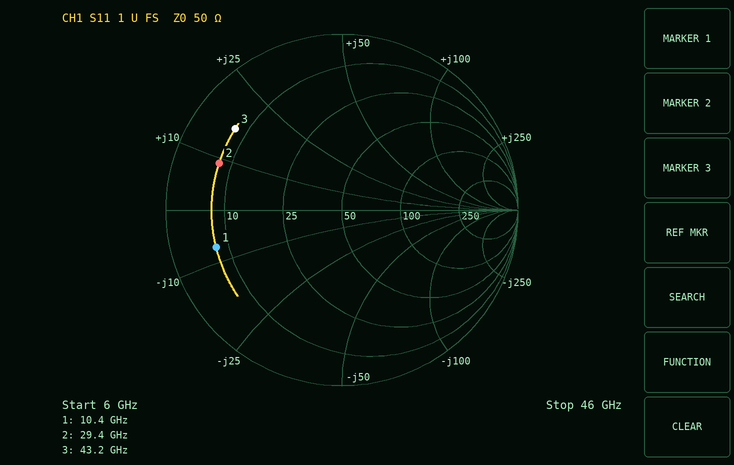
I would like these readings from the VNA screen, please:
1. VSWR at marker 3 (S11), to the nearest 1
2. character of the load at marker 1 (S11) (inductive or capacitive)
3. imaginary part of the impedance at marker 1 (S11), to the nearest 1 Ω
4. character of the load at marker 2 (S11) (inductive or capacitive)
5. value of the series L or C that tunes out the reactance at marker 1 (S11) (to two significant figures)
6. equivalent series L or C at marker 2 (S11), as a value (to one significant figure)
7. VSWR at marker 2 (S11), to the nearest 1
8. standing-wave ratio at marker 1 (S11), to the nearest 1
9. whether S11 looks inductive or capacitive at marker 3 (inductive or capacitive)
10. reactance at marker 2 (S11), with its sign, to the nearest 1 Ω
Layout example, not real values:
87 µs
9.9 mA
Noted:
7
capacitive
-7 Ω
inductive
110 pH
50 pH
7
7
inductive
+9 Ω
